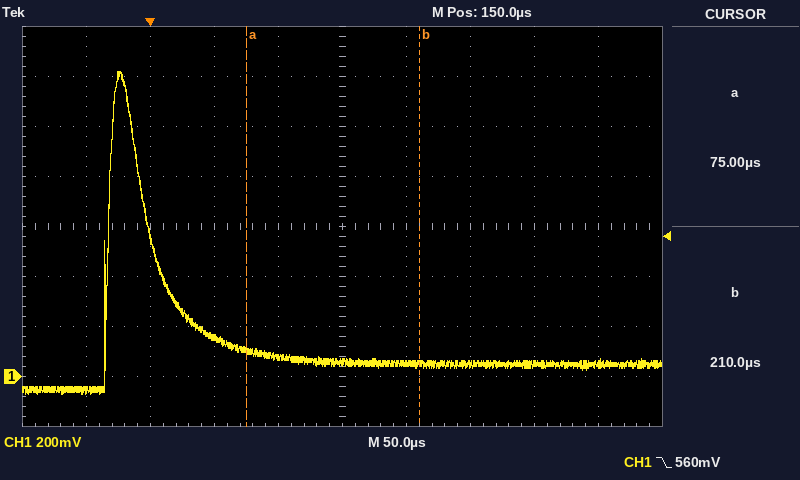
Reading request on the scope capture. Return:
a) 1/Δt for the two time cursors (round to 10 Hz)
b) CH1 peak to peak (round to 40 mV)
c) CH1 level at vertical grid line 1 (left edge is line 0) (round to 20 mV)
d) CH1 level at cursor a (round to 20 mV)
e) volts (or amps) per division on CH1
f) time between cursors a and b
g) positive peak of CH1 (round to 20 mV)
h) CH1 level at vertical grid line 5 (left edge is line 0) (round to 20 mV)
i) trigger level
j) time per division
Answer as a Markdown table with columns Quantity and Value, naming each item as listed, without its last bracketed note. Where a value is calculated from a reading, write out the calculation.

| Quantity | Value |
|---|---|
| 1/Δt for the two time cursors | 1 / 135 µs ≈ 7.41 kHz |
| CH1 peak to peak | 1.28 V |
| CH1 level at vertical grid line 1 (left edge is line 0) | -60 mV |
| CH1 level at cursor a | 100 mV |
| volts (or amps) per division on CH1 | 200 mV |
| time between cursors a and b | 210 µs − (75 µs) = 135 µs |
| positive peak of CH1 | 1.22 V |
| CH1 level at vertical grid line 5 (left edge is line 0) | 60 mV |
| trigger level | 560 mV |
| time per division | 50 µs |
